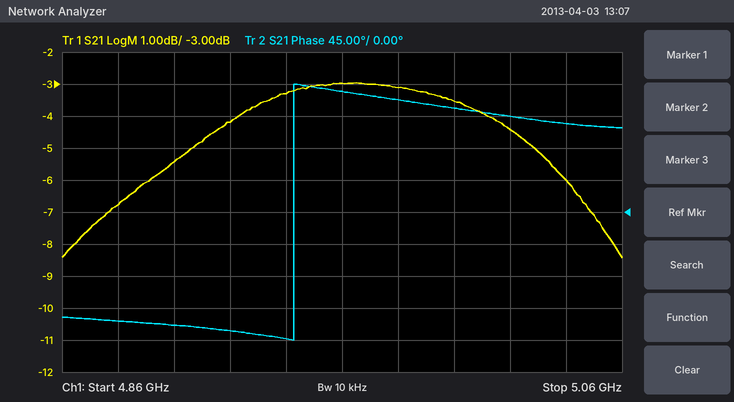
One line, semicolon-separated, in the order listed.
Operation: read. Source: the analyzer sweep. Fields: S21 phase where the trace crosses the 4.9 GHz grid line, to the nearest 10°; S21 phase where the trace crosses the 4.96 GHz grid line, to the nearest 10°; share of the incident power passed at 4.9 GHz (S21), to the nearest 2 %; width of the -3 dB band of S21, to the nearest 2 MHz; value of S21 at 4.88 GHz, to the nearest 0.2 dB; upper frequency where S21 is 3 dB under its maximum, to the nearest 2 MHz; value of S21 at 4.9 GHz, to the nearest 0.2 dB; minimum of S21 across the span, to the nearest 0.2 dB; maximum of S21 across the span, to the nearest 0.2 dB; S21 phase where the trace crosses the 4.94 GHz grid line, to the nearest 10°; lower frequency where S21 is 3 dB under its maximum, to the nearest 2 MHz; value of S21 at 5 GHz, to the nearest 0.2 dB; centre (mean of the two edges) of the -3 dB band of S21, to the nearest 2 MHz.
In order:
-160°; 170°; 28 %; 148 MHz; -6.8 dB; 5.040 GHz; -5.4 dB; -8.4 dB; -3.0 dB; -180°; 4.892 GHz; -3.6 dB; 4.966 GHz
